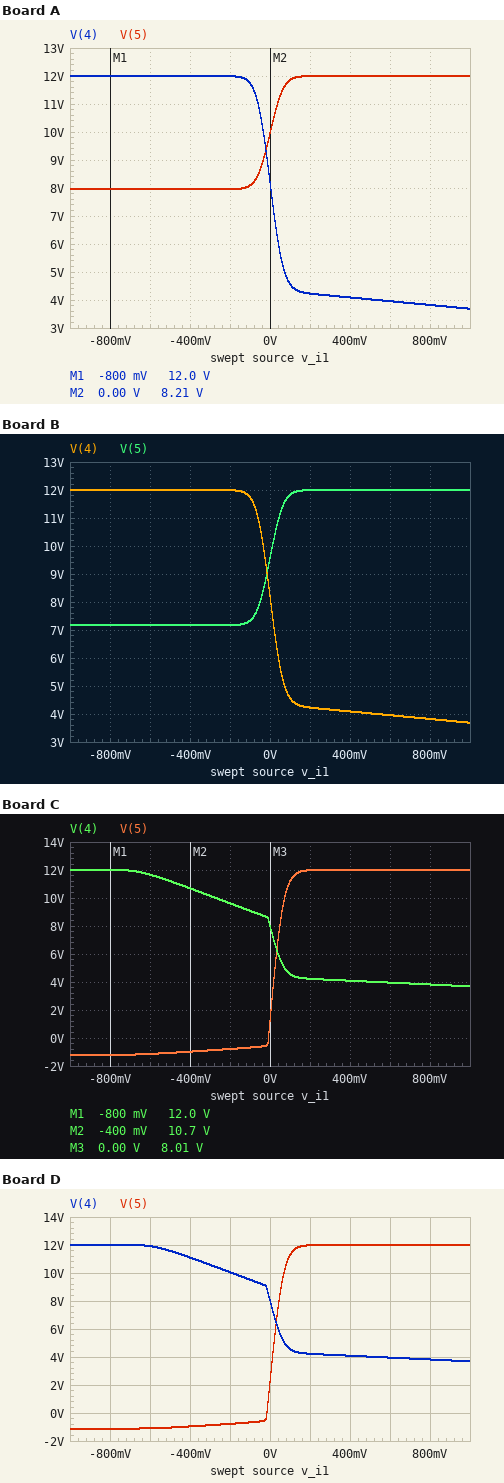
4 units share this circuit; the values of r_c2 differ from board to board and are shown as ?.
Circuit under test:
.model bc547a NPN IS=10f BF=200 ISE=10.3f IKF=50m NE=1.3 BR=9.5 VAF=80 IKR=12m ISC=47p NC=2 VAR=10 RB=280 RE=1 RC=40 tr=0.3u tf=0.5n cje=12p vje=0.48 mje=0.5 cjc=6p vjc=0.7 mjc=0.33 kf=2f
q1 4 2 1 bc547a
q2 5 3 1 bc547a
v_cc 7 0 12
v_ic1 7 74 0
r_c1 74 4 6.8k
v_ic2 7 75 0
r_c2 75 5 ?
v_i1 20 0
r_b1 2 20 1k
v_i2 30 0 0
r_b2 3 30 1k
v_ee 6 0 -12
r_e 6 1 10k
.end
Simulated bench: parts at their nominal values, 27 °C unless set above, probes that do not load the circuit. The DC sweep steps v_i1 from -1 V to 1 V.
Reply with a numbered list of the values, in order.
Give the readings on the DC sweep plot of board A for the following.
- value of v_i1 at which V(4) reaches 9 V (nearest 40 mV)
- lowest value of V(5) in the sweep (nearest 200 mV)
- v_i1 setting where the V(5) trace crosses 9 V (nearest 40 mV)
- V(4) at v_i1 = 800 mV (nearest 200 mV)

1. 0 V
2. 8.0 V
3. -40 mV
4. 3.8 V
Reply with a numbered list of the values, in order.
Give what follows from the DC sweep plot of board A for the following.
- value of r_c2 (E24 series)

1. 3.6 kΩ
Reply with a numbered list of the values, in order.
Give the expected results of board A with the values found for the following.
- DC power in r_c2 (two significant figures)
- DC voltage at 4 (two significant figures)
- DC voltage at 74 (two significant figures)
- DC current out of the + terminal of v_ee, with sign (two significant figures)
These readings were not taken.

1. 1.2 mW
2. 8.2 V
3. 12 V
4. -1.1 mA
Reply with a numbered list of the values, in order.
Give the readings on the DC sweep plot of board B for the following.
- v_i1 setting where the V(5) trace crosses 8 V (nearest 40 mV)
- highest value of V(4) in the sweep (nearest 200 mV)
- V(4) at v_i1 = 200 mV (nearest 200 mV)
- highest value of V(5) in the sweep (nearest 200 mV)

1. -40 mV
2. 12.0 V
3. 4.2 V
4. 12.0 V
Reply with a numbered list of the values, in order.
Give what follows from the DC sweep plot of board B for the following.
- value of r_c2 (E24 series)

1. 4.3 kΩ
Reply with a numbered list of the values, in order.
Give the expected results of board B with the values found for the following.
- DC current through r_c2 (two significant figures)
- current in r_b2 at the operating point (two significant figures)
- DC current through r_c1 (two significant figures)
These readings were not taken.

1. 570 µA
2. 4.6 µA
3. 560 µA
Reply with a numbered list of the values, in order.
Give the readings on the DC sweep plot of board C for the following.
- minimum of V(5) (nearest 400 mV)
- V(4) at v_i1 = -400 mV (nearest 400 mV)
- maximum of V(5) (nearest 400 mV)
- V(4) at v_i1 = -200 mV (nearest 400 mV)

1. -1.2 V
2. 10.8 V
3. 12.0 V
4. 9.6 V
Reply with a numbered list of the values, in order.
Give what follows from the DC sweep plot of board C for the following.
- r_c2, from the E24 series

1. 20 kΩ
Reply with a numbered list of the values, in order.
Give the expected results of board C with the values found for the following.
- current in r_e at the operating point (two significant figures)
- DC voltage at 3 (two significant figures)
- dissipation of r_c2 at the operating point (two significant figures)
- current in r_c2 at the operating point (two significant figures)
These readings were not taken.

1. 1.1 mA
2. -4.8 mV
3. 5.8 mW
4. 540 µA
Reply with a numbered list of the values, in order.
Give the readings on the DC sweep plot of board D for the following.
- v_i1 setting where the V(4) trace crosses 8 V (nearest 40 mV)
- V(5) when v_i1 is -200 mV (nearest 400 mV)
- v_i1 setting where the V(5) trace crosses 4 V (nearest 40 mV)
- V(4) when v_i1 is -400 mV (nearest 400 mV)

1. 0 V
2. -800 mV
3. 0 V
4. 11.2 V
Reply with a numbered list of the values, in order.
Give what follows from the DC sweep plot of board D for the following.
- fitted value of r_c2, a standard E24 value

1. 18 kΩ
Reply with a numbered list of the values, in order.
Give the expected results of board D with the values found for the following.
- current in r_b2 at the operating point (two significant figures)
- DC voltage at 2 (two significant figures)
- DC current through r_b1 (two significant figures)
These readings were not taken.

1. 4.8 µA
2. -4.8 mV
3. 4.8 µA
